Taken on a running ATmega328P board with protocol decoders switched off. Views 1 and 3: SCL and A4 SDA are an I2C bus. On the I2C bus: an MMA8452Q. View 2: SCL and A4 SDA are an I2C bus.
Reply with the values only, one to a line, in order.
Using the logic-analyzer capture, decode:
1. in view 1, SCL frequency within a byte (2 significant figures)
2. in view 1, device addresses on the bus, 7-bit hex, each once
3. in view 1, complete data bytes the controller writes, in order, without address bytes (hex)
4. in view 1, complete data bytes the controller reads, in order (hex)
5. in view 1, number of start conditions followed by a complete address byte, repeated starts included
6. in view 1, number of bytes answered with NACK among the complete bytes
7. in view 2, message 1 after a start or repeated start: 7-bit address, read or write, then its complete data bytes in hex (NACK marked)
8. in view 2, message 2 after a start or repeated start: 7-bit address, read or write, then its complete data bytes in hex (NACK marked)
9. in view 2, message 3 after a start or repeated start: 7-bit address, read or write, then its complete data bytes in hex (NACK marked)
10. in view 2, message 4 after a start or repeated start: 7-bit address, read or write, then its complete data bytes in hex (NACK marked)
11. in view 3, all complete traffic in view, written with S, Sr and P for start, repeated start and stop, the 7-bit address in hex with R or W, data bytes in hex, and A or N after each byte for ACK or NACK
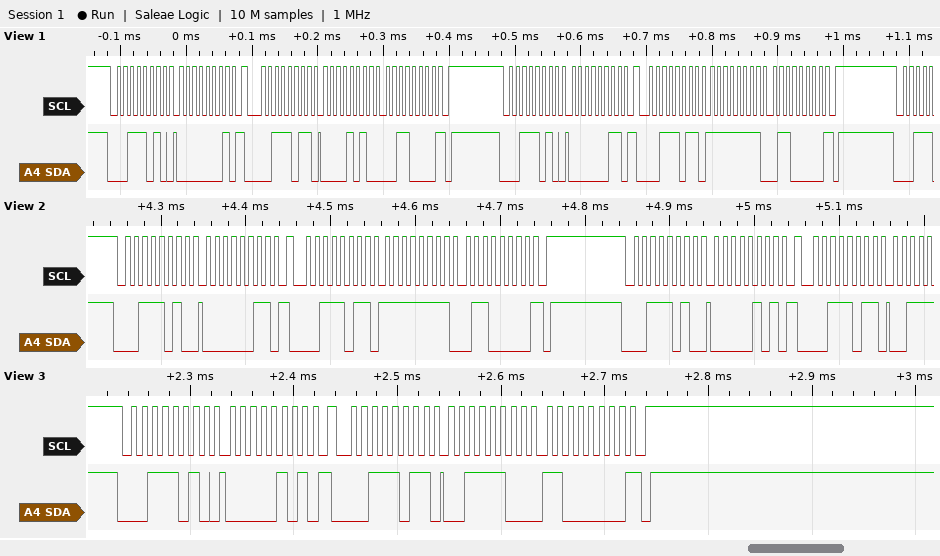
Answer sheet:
100 kHz
0x1D
01 03
0A 30 FF 60
4
2
0x1D write: 03
0x1D read: FF 60 NACK
0x1D write: 05
0x1D read
S 1DW A 05 A Sr 1DR A 3C A C0 N P
